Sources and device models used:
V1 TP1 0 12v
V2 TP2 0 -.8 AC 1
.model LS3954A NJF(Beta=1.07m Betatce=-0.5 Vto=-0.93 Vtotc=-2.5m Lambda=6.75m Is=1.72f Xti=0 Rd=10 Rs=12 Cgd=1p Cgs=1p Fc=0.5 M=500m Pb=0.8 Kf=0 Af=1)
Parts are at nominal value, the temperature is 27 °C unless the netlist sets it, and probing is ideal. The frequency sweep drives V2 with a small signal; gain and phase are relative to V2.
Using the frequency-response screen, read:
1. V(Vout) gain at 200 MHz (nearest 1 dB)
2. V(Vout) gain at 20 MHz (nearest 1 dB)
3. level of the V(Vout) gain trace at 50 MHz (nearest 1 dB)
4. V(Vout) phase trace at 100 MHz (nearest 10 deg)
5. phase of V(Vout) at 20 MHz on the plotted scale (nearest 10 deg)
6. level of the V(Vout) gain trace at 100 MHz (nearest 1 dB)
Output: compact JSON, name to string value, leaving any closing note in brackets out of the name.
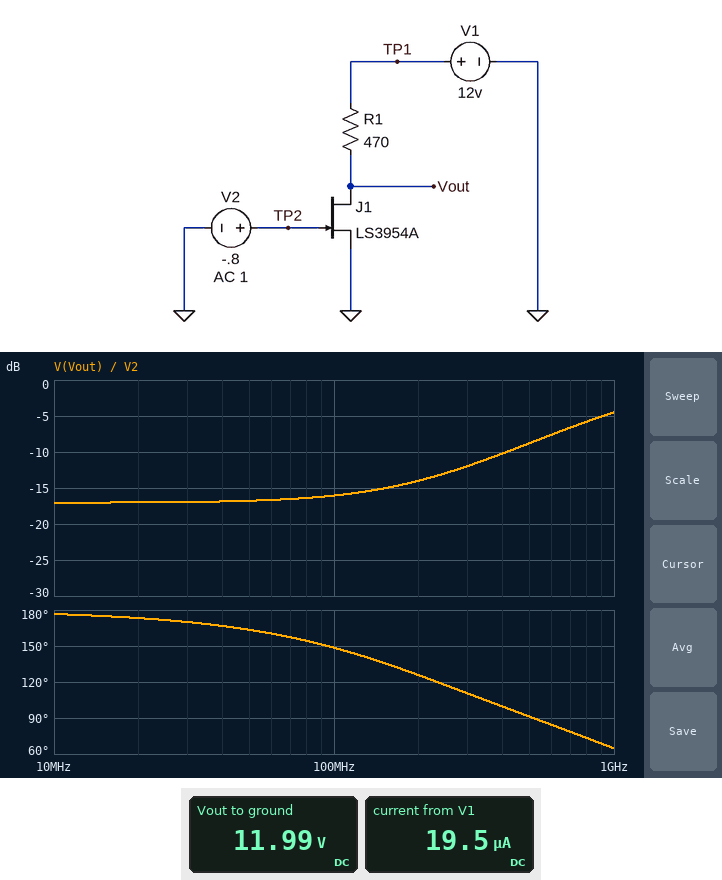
{"V(Vout) gain at 200 MHz": "-14 dB", "V(Vout) gain at 20 MHz": "-17 dB", "level of the V(Vout) gain trace at 50 MHz": "-17 dB", "V(Vout) phase trace at 100 MHz": "150 deg", "phase of V(Vout) at 20 MHz on the plotted scale": "170 deg", "level of the V(Vout) gain trace at 100 MHz": "-16 dB"}
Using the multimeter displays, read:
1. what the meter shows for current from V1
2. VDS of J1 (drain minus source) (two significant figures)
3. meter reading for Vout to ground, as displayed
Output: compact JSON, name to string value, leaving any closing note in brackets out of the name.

{"what the meter shows for current from V1": "19.5 µA", "VDS of J1 (drain minus source)": "12 V", "meter reading for Vout to ground, as displayed": "11.99 V"}
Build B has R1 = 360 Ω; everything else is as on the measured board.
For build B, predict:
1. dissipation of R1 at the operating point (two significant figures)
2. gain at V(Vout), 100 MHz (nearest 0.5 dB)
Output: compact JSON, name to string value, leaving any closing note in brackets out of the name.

{"dissipation of R1 at the operating point": "140 nW", "gain at V(Vout), 100 MHz": "-18.5 dB"}
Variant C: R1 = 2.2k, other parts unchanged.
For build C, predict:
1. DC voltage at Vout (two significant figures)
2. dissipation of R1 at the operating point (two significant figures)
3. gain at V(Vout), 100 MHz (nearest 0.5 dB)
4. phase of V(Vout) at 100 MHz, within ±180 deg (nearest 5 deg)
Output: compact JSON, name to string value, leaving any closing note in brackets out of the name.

{"DC voltage at Vout": "12 V", "dissipation of R1 at the operating point": "830 nW", "gain at V(Vout), 100 MHz": "-3.0 dB", "phase of V(Vout) at 100 MHz, within ±180 deg": "135 deg"}
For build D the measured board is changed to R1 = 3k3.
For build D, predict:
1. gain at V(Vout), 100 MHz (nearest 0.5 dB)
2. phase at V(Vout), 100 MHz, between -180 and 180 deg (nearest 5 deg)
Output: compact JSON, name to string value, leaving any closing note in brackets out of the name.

{"gain at V(Vout), 100 MHz": "0 dB", "phase at V(Vout), 100 MHz, between -180 and 180 deg": "125 deg"}
